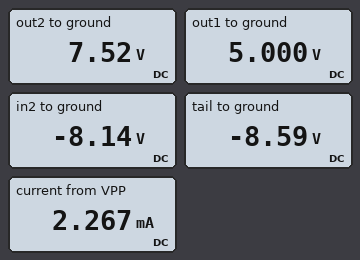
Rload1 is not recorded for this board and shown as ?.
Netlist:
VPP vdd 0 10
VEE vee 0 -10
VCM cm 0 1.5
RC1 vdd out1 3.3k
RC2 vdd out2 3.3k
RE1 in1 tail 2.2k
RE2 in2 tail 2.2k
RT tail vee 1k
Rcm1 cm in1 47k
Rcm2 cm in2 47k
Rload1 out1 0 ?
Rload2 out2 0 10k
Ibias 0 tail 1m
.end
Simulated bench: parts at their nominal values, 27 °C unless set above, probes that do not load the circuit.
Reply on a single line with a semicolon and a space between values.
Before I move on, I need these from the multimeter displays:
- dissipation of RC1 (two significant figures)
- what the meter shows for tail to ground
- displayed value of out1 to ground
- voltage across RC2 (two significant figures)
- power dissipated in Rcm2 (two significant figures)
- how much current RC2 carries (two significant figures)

7.6 mW; -8.59 V; 5.000 V; 2.5 V; 2.0 mW; 750 µA
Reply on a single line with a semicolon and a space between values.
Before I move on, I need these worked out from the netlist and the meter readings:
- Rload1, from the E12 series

3.3 kΩ
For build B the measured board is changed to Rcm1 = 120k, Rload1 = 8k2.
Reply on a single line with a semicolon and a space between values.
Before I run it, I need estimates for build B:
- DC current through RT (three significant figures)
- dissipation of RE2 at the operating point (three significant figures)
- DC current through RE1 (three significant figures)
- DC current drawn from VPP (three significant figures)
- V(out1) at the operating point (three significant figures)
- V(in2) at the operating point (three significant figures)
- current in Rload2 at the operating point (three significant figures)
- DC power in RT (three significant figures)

1.29 mA; 94.7 µW; 83.5 µA; 1.62 mA; 7.13 V; -8.25 V; 752 µA; 1.67 mW
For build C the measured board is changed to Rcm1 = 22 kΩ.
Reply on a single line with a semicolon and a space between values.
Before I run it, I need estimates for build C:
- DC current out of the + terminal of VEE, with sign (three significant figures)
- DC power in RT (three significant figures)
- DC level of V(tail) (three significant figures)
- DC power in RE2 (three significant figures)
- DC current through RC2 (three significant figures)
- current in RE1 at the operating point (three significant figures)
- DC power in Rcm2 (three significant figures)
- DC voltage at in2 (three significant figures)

-1.61 mA; 2.59 mW; -8.39 V; 88.9 µW; 752 µA; 409 µA; 1.90 mW; -7.95 V
